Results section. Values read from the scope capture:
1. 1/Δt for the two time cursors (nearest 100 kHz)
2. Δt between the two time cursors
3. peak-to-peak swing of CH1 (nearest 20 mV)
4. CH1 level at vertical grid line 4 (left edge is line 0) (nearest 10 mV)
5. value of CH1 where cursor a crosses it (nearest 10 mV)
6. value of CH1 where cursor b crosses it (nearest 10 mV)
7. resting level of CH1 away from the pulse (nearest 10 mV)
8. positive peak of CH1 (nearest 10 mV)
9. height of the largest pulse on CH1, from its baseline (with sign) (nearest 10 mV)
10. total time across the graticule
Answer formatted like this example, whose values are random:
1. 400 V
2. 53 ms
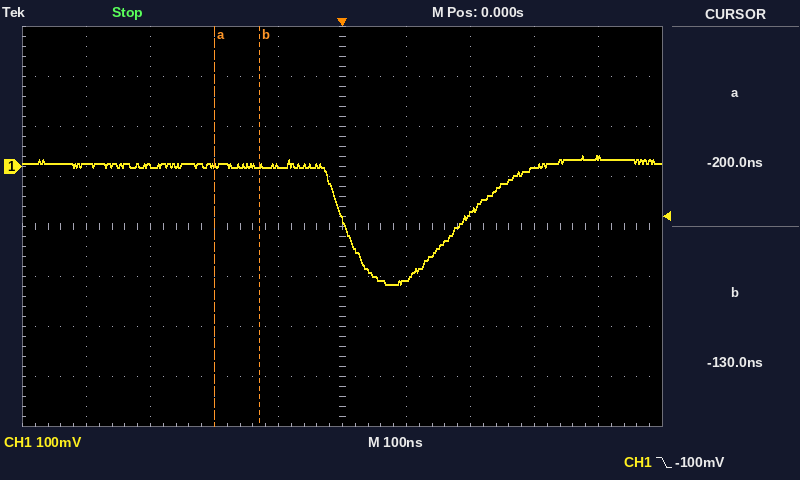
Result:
1. 14.3 MHz
2. 70 ns
3. 260 mV
4. 0 mV
5. 0 mV
6. 0 mV
7. 0 mV
8. 20 mV
9. -240 mV
10. 1 µs
